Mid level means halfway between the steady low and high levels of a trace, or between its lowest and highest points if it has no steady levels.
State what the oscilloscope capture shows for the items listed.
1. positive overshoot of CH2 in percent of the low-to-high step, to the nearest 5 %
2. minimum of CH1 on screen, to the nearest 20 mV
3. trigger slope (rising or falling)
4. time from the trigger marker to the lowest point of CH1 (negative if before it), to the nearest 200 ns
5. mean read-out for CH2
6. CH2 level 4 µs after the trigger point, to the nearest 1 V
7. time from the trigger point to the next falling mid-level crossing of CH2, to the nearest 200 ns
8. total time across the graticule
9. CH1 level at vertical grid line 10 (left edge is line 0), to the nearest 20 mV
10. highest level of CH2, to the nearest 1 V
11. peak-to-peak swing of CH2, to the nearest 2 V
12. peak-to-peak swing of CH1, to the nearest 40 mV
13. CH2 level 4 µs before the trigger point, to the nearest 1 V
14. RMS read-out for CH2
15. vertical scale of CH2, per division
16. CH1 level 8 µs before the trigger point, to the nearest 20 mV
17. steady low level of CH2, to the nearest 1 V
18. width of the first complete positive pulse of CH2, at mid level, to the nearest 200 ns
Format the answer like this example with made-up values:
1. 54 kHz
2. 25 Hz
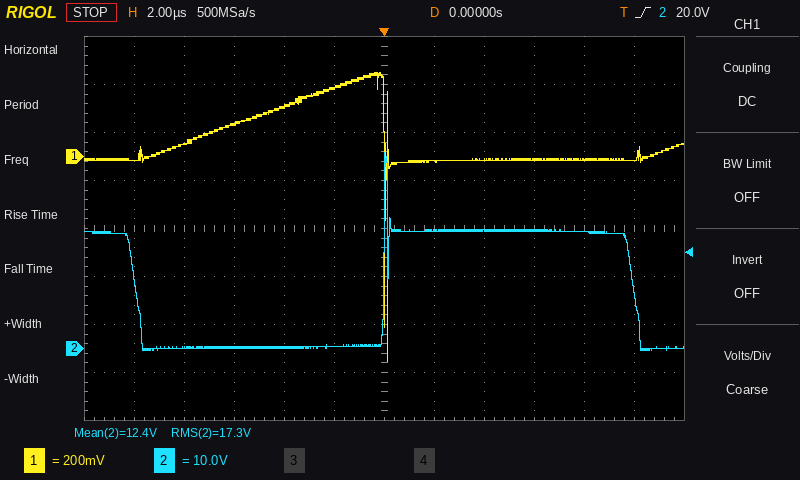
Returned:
1. 65 %
2. -860 mV
3. rising
4. +200 ns
5. 12.4 V
6. 25 V
7. 10.0 µs
8. 24 µs
9. -20 mV
10. 41 V
11. 42 V
12. 1.20 V
13. 0 V
14. 17.3 V
15. 10 V
16. 60 mV
17. 0 V
18. 10.0 µs
